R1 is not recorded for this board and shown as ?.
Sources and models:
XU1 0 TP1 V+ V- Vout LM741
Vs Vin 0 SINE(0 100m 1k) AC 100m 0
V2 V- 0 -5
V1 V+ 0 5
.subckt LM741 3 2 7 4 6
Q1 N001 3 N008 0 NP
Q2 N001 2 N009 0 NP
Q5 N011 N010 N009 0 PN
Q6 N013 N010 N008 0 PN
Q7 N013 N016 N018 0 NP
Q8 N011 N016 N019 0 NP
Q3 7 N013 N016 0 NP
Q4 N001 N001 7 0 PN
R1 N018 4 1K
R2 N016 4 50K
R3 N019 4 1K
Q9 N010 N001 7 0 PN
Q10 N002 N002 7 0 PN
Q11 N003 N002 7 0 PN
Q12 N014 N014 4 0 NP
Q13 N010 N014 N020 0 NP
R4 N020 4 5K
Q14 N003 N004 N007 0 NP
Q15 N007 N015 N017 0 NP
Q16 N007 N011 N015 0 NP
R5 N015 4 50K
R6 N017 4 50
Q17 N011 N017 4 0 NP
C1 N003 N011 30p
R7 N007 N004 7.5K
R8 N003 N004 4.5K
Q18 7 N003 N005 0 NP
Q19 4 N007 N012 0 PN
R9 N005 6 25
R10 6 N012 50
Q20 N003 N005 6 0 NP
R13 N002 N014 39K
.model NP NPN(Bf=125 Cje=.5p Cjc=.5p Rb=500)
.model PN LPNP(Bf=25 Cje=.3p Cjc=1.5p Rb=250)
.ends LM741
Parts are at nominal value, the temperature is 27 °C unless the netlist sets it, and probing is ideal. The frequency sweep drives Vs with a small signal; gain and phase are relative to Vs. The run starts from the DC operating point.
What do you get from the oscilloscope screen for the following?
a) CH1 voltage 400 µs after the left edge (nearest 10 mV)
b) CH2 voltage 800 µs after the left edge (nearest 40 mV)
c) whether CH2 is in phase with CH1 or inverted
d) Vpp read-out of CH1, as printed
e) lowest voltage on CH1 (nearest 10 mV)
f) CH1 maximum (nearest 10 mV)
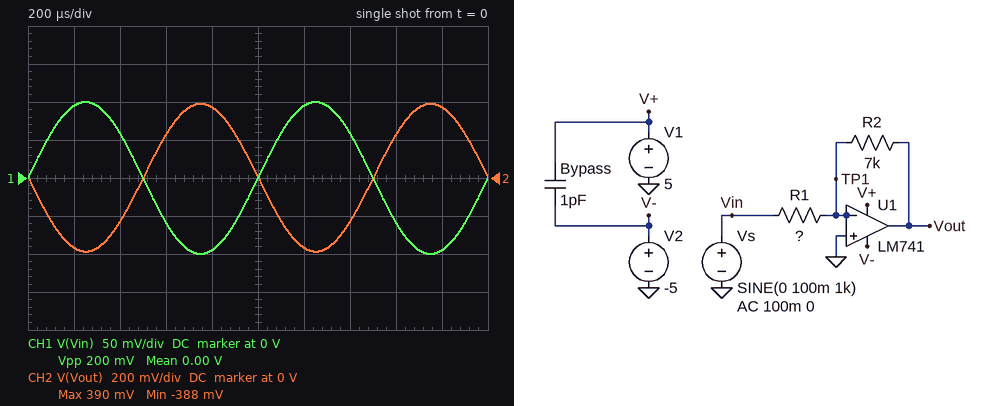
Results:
60 mV
360 mV
inverted
200 mV
-100 mV
100 mV
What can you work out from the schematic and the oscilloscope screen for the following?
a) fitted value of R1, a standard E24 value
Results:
1.8 kΩ
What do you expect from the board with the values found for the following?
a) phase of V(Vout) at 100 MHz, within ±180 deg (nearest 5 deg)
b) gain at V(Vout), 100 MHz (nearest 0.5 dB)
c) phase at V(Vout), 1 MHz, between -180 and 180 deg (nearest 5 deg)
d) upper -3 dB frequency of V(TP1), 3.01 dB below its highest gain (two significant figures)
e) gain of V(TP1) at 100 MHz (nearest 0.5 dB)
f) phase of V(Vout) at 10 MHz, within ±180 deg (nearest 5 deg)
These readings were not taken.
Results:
-75 deg
-19.0 dB
10 deg
86 MHz
-4.0 dB
-35 deg
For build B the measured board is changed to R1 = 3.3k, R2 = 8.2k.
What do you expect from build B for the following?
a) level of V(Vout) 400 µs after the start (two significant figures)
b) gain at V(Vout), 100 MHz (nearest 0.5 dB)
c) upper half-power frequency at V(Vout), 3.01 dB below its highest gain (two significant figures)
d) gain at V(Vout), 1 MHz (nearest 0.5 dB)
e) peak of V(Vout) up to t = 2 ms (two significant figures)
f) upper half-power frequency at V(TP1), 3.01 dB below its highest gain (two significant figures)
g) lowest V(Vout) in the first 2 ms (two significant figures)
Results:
-150 mV
-22.5 dB
65 kHz
-3.5 dB
250 mV
37 MHz
-250 mV
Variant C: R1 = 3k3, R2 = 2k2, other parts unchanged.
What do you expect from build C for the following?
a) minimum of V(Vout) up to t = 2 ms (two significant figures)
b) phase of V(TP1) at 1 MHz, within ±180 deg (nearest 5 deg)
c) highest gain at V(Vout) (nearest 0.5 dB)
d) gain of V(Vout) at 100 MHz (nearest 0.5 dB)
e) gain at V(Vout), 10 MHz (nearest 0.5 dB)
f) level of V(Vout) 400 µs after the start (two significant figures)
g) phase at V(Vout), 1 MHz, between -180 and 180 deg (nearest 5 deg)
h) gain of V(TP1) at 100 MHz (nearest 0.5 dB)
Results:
-66 mV
0 deg
-2.0 dB
-16.0 dB
-3.0 dB
-39 mV
5 deg
-9.0 dB
